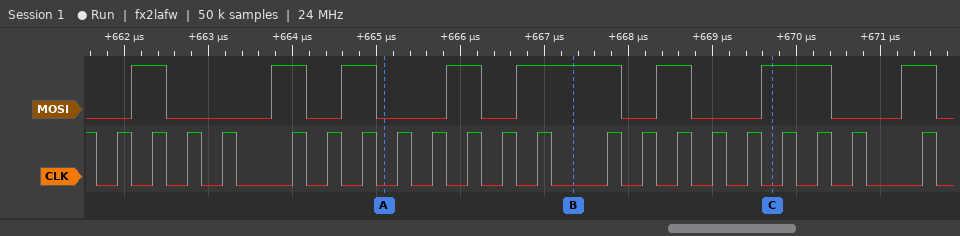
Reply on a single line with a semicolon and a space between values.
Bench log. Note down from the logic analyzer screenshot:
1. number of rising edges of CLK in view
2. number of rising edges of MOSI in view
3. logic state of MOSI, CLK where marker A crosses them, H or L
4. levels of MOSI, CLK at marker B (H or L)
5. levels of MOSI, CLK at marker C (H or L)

21; 8; MOSI=L, CLK=L; MOSI=H, CLK=L; MOSI=H, CLK=L
